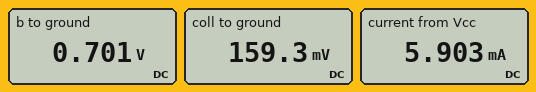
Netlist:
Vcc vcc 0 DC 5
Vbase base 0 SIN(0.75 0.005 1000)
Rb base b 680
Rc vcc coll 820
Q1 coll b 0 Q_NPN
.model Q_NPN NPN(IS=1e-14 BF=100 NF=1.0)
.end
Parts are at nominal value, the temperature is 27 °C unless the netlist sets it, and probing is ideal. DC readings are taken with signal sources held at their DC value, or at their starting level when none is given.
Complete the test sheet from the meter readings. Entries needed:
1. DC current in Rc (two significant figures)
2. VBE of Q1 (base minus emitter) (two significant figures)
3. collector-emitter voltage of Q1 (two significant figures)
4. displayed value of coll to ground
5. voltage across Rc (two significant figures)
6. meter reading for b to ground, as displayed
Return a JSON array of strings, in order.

["5.9 mA", "700 mV", "160 mV", "159.3 mV", "4.8 V", "0.701 V"]
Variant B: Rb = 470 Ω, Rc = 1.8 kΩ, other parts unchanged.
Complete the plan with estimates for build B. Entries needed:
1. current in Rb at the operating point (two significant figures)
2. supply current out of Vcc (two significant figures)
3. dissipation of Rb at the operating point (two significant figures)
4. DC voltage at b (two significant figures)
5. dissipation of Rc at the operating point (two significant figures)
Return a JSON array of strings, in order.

["140 µA", "2.7 mA", "9.5 µW", "680 mV", "13 mW"]
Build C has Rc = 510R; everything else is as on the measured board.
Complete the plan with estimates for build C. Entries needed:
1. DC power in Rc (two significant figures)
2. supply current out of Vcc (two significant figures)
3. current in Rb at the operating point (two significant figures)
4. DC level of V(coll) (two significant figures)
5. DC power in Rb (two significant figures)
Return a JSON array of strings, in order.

["23 mW", "6.7 mA", "67 µA", "1.6 V", "3.1 µW"]
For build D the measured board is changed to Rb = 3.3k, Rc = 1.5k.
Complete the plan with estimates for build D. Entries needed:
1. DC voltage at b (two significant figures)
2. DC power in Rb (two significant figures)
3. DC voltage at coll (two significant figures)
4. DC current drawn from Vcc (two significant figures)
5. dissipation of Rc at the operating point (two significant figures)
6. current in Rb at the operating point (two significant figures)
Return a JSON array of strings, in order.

["680 mV", "1.7 µW", "1.6 V", "2.2 mA", "7.5 mW", "22 µA"]
